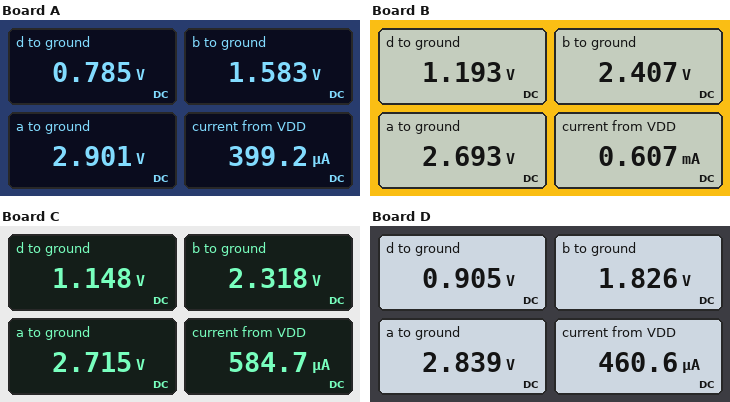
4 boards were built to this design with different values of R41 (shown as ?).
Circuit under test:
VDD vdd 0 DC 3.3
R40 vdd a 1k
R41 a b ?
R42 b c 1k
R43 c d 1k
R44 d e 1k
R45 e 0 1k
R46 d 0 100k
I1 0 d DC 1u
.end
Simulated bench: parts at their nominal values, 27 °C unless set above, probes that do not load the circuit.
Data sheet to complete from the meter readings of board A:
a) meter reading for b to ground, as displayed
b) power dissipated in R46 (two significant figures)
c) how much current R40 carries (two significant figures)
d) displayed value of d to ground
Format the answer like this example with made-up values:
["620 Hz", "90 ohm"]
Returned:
["1.583 V", "6.2 µW", "400 µA", "0.785 V"]
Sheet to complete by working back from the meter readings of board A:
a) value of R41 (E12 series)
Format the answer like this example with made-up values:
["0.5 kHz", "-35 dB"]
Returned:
["3.3 kΩ"]
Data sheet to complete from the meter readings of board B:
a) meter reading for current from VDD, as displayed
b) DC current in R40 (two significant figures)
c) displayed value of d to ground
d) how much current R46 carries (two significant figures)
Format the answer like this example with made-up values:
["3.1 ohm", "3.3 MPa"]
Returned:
["0.607 mA", "610 µA", "1.193 V", "12 µA"]
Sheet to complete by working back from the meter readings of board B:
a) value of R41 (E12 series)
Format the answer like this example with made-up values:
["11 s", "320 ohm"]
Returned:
["470 Ω"]
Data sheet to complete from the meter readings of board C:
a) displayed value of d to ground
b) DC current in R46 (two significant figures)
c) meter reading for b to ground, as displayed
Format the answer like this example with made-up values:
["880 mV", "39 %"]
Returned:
["1.148 V", "11 µA", "2.318 V"]
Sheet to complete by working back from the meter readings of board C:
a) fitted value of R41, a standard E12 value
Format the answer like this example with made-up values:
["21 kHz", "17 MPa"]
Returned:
["680 Ω"]
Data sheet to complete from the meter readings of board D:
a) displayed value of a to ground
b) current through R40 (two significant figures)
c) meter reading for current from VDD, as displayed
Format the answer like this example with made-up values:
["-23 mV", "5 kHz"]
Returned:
["2.839 V", "460 µA", "460.6 µA"]
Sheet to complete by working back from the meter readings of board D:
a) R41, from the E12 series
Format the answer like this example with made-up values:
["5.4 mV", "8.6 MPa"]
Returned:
["2.2 kΩ"]
